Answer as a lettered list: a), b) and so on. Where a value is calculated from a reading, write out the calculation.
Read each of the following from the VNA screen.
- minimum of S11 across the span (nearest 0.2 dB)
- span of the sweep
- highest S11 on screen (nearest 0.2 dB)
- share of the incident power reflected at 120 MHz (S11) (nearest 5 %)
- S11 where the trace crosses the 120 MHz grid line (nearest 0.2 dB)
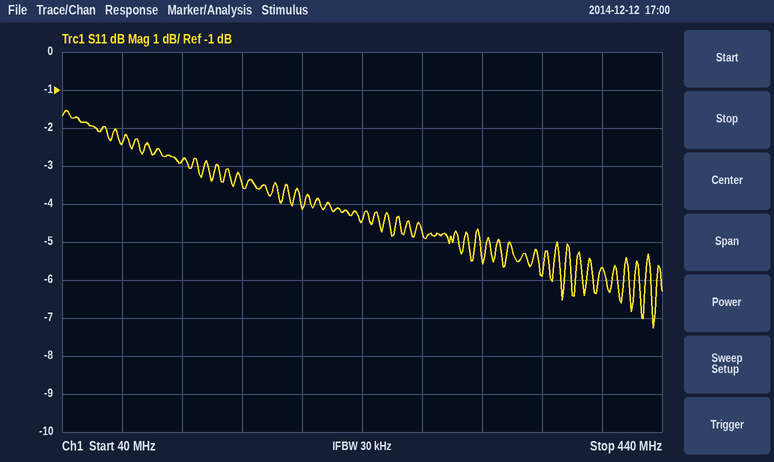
a) -7.2 dB
b) 400 MHz
c) -1.6 dB
d) 10^(-2.8/10) ≈ 52.5 %, so 50 % to the nearest 5 %
e) -2.8 dB
